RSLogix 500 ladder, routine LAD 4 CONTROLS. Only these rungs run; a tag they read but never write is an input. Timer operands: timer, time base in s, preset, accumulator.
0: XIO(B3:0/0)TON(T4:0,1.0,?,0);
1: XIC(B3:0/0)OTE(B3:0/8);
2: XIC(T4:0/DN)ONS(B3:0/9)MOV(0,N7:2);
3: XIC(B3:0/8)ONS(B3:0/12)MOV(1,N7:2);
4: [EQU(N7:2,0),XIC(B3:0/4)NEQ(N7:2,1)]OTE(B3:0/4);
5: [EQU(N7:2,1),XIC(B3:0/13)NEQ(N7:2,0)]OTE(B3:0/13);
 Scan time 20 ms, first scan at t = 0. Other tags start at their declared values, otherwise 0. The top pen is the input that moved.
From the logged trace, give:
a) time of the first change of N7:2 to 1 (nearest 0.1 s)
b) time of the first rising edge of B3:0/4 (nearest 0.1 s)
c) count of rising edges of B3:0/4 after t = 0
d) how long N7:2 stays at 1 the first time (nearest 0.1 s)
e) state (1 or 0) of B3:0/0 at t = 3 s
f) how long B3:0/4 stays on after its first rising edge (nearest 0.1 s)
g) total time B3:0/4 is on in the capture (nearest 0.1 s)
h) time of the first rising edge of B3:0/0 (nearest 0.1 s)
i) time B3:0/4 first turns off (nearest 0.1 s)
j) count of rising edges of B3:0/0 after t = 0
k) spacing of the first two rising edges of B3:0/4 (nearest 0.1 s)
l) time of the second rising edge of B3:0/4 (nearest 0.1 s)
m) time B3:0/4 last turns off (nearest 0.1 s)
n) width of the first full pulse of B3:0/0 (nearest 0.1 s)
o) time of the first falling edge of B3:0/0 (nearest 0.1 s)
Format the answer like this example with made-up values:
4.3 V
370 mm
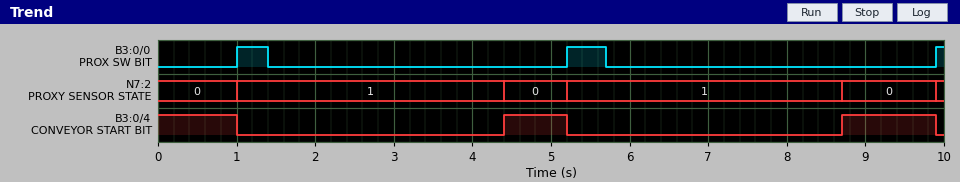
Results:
1.0 s
4.4 s
2
3.4 s
0
0.8 s
3.0 s
1.0 s
1.0 s
3
4.3 s
8.7 s
9.9 s
0.4 s
1.4 s
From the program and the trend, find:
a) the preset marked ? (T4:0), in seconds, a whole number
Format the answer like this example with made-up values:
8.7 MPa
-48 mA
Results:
3 s
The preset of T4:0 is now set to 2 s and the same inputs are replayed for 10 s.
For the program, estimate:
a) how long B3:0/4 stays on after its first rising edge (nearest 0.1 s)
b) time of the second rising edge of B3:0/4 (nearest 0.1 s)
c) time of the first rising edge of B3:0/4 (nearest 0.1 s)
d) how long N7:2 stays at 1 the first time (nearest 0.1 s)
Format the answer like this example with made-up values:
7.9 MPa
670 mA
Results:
1.8 s
7.7 s
3.4 s
2.4 s
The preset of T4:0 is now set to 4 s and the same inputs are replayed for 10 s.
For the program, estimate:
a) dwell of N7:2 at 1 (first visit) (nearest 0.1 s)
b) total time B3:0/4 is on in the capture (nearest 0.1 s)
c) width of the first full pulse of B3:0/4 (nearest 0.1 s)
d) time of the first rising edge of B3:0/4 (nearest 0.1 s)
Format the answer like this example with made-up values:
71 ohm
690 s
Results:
8.7 s
1.2 s
0.2 s
9.7 s
